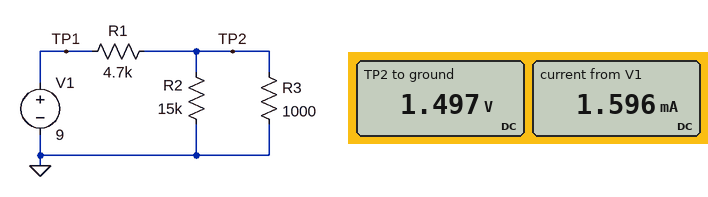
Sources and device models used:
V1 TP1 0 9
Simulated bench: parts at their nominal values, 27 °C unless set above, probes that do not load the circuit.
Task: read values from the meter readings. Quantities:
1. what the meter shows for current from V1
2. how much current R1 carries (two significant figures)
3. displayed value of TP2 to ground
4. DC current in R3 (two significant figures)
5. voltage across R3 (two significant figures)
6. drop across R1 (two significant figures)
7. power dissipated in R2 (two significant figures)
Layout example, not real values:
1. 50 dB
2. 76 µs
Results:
1. 1.596 mA
2. 1.6 mA
3. 1.497 V
4. 1.5 mA
5. 1.5 V
6. 7.5 V
7. 150 µW
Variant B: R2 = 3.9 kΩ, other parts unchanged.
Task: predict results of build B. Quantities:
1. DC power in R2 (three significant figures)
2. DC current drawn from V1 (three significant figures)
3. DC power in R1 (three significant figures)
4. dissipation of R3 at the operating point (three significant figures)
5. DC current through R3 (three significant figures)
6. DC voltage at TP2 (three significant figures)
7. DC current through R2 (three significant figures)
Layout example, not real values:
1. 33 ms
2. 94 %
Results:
1. 436 µW
2. 1.64 mA
3. 12.6 mW
4. 1.70 mW
5. 1.30 mA
6. 1.30 V
7. 334 µA
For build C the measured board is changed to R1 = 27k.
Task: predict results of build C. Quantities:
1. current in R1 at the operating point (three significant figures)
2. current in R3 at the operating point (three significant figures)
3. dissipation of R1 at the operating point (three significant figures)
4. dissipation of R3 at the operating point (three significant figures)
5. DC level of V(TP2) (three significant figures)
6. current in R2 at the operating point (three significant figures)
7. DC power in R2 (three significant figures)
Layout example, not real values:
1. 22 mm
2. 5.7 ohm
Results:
1. 322 µA
2. 302 µA
3. 2.80 mW
4. 91.2 µW
5. 302 mV
6. 20.1 µA
7. 6.08 µW
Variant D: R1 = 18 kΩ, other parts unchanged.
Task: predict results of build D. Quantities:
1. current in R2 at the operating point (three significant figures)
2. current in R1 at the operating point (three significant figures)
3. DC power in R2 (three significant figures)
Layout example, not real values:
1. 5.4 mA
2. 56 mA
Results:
1. 29.7 µA
2. 475 µA
3. 13.2 µW
